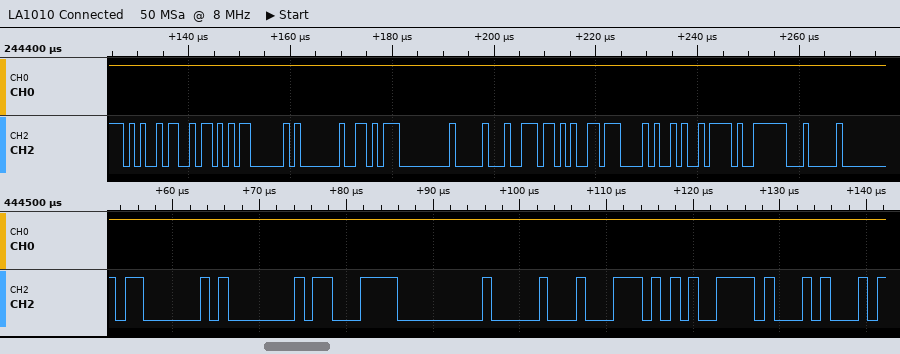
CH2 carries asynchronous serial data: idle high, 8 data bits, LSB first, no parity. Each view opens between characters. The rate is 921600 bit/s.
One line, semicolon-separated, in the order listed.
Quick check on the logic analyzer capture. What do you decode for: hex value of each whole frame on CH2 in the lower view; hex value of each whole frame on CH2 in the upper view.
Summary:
03, 01, E3, 00, 10, 5C, 79, 14; A5, 5A, 03, 01, D6, 00, 10, 6E, D9, 28, E9, F9, 04
